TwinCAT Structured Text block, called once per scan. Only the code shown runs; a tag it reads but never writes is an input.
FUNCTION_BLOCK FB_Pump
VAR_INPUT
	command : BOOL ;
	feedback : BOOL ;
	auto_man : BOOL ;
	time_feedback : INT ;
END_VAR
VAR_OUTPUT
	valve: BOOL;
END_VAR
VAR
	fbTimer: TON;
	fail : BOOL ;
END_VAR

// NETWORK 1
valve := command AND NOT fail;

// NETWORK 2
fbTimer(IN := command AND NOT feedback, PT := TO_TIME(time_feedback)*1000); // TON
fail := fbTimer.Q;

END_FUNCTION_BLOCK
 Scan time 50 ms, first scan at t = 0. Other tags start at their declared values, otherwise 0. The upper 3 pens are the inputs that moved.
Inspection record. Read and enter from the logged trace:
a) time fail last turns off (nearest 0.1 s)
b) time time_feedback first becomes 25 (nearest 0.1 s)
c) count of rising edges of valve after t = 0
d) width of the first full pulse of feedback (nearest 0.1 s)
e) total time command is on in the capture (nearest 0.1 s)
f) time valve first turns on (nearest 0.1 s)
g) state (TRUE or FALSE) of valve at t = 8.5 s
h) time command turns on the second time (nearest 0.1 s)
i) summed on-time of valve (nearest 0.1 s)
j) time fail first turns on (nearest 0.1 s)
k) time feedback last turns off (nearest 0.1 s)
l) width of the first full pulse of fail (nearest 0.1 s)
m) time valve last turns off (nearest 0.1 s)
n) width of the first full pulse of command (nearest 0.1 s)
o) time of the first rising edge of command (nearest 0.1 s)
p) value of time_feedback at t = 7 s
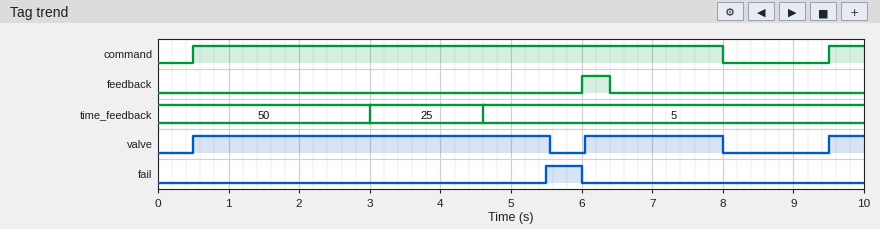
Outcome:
6.0 s
3.0 s
3
0.4 s
8.0 s
0.5 s
FALSE
9.5 s
7.5 s
5.5 s
6.4 s
0.5 s
8.0 s
7.5 s
0.5 s
5
